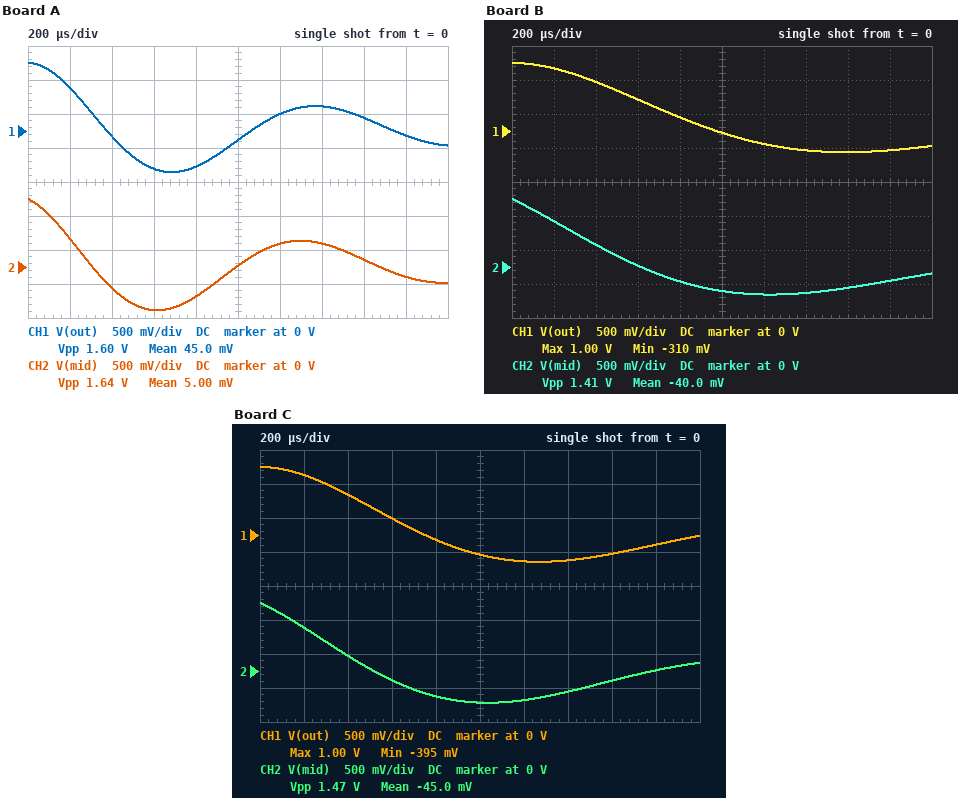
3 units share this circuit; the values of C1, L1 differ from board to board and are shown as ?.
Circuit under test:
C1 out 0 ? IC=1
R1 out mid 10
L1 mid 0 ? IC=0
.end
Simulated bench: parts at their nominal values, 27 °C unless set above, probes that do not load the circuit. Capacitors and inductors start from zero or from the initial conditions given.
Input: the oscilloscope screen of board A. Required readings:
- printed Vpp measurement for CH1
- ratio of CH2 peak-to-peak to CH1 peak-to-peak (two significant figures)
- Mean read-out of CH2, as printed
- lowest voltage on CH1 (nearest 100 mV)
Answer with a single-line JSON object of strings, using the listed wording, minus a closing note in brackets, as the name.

{"printed Vpp measurement for CH1": "1.60 V", "ratio of CH2 peak-to-peak to CH1 peak-to-peak": "1.0", "Mean read-out of CH2, as printed": "5.00 mV", "lowest voltage on CH1": "-600 mV"}
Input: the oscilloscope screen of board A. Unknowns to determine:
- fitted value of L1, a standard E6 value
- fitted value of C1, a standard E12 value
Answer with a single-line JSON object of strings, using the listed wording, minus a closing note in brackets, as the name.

{"fitted value of L1, a standard E6 value": "6.8 mH", "fitted value of C1, a standard E12 value": "6.8 µF"}
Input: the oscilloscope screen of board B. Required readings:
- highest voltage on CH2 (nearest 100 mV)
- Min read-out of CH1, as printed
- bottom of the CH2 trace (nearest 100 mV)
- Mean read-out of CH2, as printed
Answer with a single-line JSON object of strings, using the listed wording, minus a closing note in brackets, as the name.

{"highest voltage on CH2": "1.0 V", "Min read-out of CH1, as printed": "-310 mV", "bottom of the CH2 trace": "-400 mV", "Mean read-out of CH2, as printed": "-40.0 mV"}
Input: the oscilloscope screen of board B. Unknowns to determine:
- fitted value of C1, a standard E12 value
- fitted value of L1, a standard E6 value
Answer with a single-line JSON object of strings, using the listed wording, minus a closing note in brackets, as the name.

{"fitted value of C1, a standard E12 value": "33 µF", "fitted value of L1, a standard E6 value": "6.8 mH"}
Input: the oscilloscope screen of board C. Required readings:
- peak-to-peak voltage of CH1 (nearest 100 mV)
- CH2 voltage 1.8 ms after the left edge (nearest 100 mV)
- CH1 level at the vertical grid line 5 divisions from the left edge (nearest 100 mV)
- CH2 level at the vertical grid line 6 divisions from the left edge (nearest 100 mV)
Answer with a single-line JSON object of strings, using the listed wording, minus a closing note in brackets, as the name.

{"peak-to-peak voltage of CH1": "1.4 V", "CH2 voltage 1.8 ms after the left edge": "0 V", "CH1 level at the vertical grid line 5 divisions from the left edge": "-300 mV", "CH2 level at the vertical grid line 6 divisions from the left edge": "-400 mV"}
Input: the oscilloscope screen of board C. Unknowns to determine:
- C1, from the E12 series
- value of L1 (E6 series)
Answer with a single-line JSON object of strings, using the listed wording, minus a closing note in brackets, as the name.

{"C1, from the E12 series": "22 µF", "value of L1": "6.8 mH"}
